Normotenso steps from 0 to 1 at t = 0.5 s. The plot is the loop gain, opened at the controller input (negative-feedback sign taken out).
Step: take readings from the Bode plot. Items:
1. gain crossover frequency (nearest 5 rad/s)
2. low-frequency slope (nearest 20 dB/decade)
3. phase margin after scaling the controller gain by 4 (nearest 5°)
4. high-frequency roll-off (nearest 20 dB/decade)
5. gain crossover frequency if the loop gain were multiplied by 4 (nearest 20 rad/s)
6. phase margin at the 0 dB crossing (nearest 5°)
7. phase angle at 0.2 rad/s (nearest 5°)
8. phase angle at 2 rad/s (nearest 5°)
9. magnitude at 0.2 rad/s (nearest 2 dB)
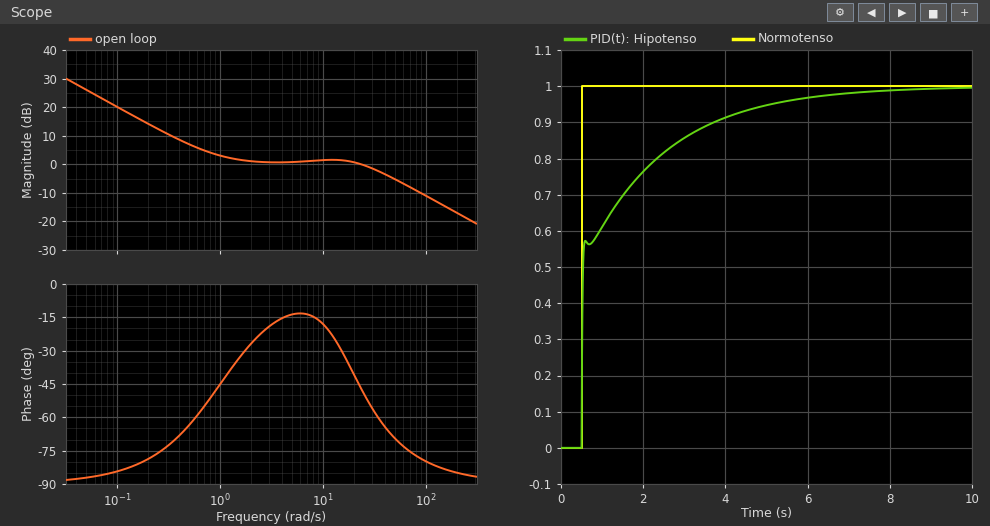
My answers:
25 rad/s
-20 dB/decade
100°
-20 dB/decade
120 rad/s
135°
-80°
-25°
14 dB
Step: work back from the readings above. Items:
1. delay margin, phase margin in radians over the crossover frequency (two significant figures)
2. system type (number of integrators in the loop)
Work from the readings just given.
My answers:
0.094 s
1
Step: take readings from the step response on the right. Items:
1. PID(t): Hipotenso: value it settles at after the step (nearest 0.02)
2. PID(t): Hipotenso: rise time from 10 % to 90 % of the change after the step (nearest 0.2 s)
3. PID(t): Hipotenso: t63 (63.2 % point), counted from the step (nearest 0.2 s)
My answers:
1.00
3.2 s
0.6 s
